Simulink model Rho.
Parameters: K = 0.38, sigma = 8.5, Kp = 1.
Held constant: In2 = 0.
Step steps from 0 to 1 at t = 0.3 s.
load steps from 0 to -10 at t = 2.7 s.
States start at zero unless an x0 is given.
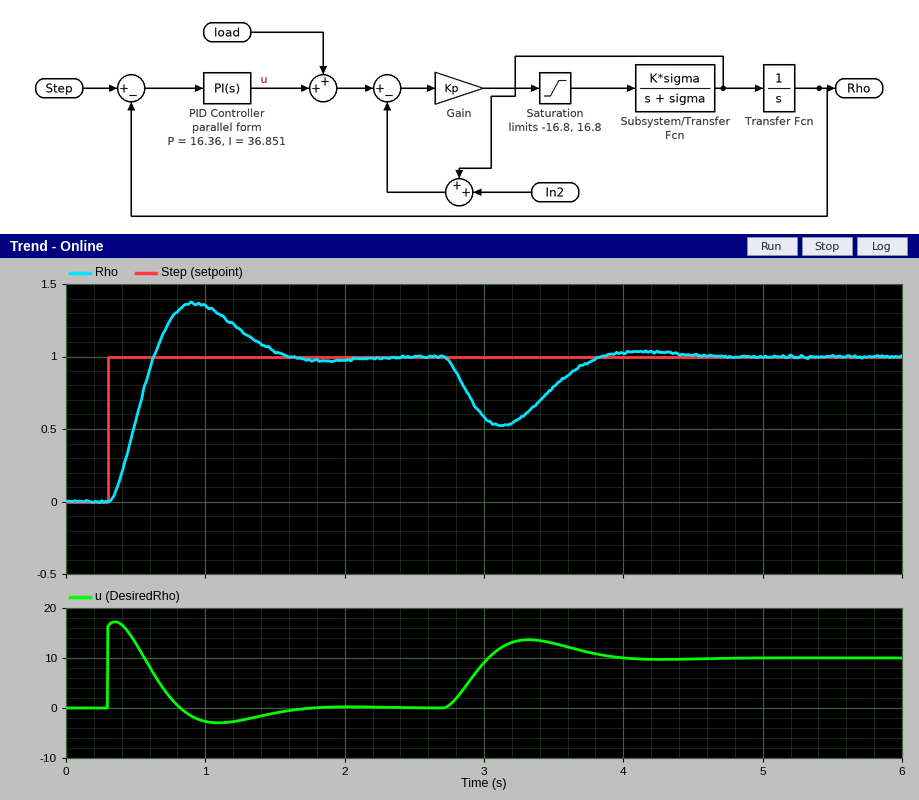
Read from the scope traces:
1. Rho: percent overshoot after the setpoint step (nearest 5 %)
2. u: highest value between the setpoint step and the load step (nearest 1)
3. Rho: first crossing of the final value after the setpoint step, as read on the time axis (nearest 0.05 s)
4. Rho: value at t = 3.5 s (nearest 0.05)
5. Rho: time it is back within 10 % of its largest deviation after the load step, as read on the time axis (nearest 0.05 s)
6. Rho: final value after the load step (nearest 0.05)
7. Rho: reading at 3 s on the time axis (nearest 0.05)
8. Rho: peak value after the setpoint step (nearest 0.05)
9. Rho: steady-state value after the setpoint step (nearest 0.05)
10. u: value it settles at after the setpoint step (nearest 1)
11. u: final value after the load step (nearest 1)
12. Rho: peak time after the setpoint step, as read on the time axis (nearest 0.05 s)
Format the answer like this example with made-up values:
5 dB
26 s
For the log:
35 %
17
0.65 s
0.80
3.75 s
1.00
0.60
1.35
1.00
0
10
0.90 s
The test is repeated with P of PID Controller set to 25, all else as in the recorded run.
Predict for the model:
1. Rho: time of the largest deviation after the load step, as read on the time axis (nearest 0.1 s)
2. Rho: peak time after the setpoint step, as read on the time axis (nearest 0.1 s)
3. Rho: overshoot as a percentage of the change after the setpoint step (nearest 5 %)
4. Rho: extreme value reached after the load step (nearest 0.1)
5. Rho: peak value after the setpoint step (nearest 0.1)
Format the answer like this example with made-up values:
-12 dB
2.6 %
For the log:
3.1 s
0.8 s
30 %
0.6
1.3
